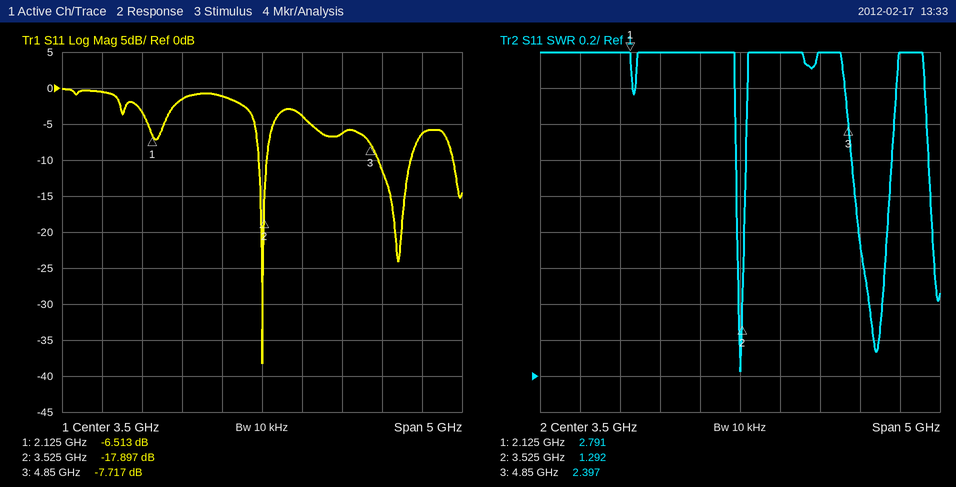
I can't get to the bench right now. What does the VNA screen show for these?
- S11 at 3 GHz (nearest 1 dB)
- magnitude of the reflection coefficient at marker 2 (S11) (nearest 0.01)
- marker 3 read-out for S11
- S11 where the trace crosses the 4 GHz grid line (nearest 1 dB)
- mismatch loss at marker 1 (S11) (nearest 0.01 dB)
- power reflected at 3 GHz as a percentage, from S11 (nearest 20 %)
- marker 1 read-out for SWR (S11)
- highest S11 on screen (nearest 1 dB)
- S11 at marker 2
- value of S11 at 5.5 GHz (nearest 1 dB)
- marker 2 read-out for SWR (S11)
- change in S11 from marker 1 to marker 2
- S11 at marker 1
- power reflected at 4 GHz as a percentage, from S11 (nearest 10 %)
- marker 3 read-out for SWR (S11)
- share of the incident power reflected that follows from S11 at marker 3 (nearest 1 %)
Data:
-1 dB
0.13
-7.717 dB
-4 dB
1.10 dB
80 %
2.791
0 dB
-17.897 dB
-6 dB
1.292
-11.384 dB
-6.513 dB
40 %
2.397
17 %
